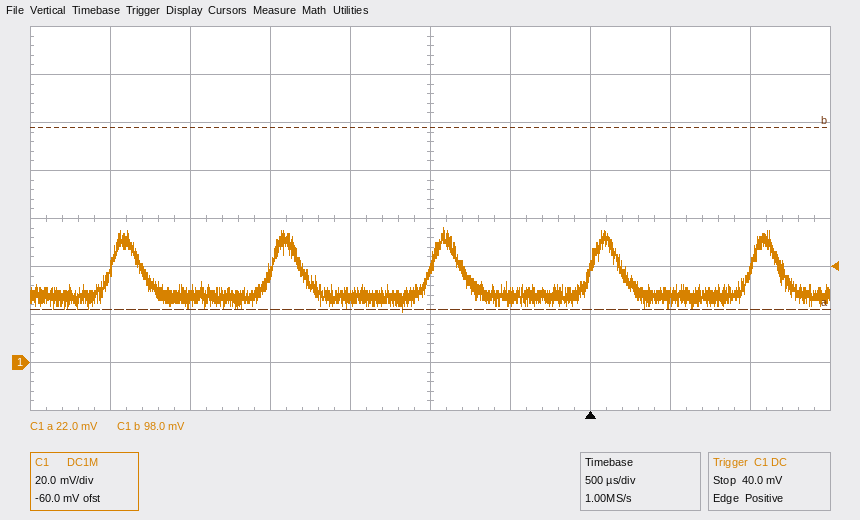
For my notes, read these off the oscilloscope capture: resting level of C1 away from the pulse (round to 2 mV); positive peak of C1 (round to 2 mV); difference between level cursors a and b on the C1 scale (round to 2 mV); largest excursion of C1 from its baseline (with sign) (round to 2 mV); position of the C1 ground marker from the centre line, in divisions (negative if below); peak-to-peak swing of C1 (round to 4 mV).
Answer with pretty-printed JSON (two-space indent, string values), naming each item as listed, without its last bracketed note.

{
  "resting level of C1 away from the pulse": "28 mV",
  "positive peak of C1": "56 mV",
  "difference between level cursors a and b on the C1 scale": "76 mV",
  "largest excursion of C1 from its baseline (with sign)": "+28 mV",
  "position of the C1 ground marker from the centre line, in divisions": "-3.0 div",
  "peak-to-peak swing of C1": "36 mV"
}
